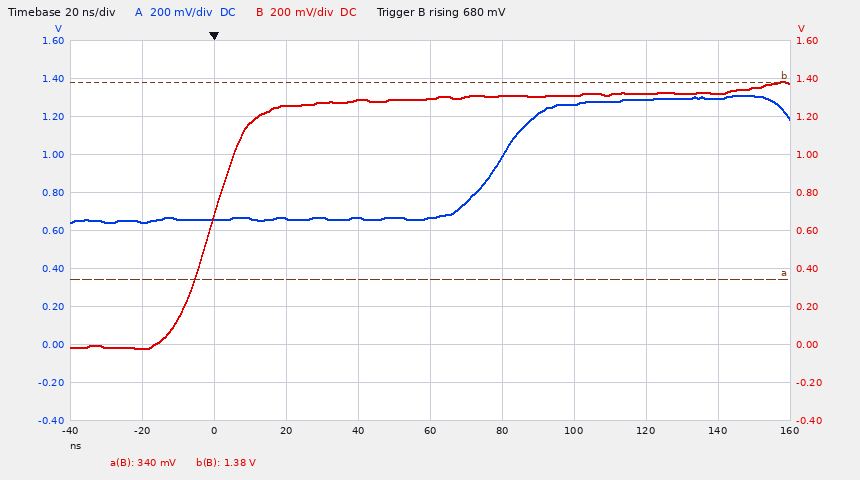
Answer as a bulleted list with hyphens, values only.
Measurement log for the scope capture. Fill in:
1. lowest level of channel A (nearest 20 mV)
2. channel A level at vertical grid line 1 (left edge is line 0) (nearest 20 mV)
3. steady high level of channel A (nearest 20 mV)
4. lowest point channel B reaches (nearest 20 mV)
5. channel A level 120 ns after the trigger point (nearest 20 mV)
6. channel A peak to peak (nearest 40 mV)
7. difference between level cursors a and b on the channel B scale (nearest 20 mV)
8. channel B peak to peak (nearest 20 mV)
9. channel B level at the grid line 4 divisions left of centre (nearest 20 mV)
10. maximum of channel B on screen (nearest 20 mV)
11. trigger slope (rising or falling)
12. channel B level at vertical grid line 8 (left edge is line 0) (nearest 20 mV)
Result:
- 640 mV
- 640 mV
- 1.30 V
- -20 mV
- 1.28 V
- 680 mV
- 1.04 V
- 1.40 V
- -20 mV
- 1.38 V
- rising
- 1.32 V
